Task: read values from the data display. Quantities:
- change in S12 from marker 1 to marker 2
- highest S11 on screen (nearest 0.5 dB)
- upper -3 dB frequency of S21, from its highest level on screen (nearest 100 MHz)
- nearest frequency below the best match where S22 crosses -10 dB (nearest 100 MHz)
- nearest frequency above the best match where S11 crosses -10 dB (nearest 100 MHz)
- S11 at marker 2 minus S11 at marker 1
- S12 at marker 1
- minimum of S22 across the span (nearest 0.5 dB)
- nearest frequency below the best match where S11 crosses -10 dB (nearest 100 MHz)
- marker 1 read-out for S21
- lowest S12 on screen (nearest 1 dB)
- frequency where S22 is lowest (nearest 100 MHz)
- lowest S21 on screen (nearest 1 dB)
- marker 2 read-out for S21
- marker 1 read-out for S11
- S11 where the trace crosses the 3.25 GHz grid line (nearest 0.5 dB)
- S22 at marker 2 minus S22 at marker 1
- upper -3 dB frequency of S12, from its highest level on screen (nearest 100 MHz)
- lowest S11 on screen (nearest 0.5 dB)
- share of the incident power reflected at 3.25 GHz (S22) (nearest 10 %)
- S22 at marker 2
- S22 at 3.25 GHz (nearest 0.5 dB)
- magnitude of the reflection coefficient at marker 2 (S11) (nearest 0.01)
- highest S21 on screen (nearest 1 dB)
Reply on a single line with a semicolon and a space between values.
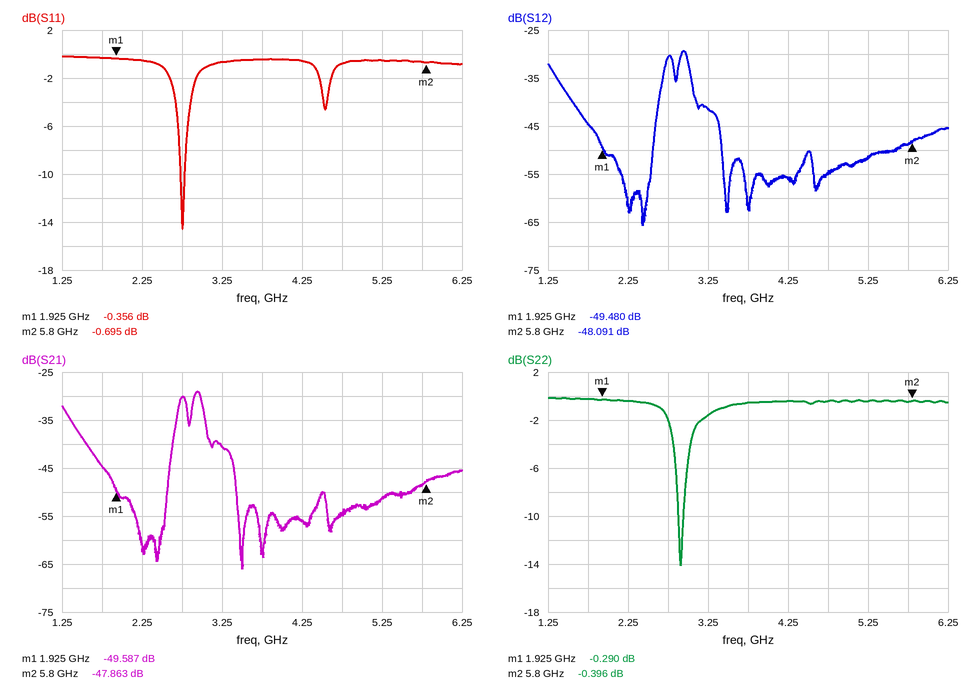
1.389 dB; 0.0 dB; 3.0 GHz; 2.9 GHz; 2.8 GHz; -0.339 dB; -49.480 dB; -14.0 dB; 2.7 GHz; -49.587 dB; -66 dB; 2.9 GHz; -66 dB; -47.863 dB; -0.356 dB; -0.5 dB; -0.106 dB; 3.0 GHz; -14.5 dB; 70 %; -0.396 dB; -1.5 dB; 0.92; -29 dB
